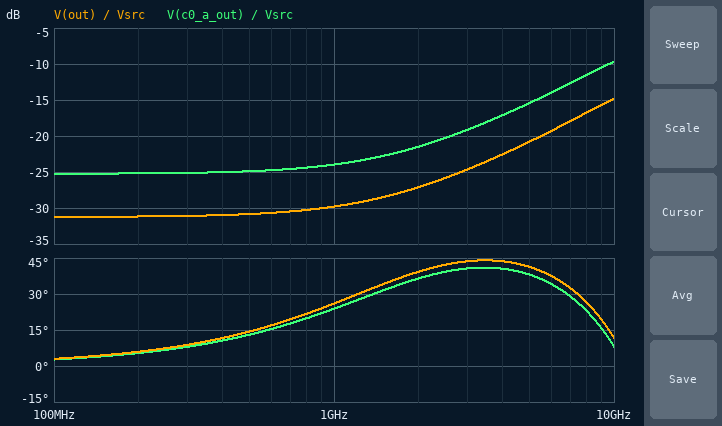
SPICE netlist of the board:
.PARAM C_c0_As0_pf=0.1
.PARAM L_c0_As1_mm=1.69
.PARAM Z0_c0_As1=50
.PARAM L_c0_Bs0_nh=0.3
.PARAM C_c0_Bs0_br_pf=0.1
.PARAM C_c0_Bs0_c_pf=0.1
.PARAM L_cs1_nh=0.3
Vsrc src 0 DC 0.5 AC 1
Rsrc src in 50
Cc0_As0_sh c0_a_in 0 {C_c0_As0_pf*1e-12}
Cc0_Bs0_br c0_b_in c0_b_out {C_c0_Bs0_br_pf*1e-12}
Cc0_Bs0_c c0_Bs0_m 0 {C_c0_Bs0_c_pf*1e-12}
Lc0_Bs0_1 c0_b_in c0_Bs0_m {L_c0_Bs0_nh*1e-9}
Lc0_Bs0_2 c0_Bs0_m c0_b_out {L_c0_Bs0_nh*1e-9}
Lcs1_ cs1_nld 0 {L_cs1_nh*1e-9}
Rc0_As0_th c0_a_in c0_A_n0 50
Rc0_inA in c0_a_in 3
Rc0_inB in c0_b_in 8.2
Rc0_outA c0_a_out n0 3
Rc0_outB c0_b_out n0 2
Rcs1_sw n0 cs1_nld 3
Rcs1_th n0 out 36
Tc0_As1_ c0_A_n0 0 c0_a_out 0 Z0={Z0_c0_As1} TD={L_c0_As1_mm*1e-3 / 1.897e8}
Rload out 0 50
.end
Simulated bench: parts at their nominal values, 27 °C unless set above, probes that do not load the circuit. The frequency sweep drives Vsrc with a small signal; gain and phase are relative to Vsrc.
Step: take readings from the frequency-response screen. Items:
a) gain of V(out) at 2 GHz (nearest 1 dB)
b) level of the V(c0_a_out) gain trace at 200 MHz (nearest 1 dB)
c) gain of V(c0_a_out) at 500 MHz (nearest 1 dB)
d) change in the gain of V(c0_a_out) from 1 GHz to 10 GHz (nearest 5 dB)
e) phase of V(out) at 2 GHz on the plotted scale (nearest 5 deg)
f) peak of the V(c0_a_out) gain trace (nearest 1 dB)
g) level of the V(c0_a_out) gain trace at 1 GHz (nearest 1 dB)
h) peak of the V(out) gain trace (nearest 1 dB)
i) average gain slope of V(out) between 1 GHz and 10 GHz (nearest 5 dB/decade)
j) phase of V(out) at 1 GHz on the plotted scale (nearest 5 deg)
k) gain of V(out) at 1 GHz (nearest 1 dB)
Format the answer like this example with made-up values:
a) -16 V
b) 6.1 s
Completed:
a) -27 dB
b) -25 dB
c) -25 dB
d) 15 dB
e) 40 deg
f) -10 dB
g) -24 dB
h) -15 dB
i) 15 dB/decade
j) 25 deg
k) -30 dB
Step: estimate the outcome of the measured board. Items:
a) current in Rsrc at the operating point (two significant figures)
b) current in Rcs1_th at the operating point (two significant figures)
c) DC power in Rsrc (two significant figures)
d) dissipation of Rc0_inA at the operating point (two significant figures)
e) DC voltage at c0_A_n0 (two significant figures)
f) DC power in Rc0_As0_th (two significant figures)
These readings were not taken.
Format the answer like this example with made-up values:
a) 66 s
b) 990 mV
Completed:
a) 8.1 mA
b) 270 µA
c) 3.3 mW
d) 4.7 µW
e) 27 mV
f) 78 µW
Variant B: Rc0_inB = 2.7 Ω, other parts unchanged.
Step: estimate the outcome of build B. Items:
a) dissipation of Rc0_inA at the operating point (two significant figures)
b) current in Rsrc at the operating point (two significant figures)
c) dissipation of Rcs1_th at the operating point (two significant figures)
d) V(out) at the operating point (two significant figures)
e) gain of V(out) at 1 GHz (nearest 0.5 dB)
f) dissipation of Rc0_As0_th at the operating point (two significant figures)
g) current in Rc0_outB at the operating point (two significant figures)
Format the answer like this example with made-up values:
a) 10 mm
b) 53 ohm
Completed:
a) 1.4 µW
b) 8.7 mA
c) 3.1 µW
d) 15 mV
e) -29.0 dB
f) 23 µW
g) 8.1 mA
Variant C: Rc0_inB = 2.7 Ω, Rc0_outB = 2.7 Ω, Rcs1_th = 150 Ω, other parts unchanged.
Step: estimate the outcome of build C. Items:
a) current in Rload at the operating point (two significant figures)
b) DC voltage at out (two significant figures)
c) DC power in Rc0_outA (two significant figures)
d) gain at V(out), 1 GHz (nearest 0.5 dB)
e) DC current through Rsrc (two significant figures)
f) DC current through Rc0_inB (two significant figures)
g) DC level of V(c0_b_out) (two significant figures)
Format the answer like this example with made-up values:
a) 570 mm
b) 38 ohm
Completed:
a) 130 µA
b) 6.4 mV
c) 1.7 µW
d) -36.5 dB
e) 8.6 mA
f) 7.9 mA
g) 47 mV
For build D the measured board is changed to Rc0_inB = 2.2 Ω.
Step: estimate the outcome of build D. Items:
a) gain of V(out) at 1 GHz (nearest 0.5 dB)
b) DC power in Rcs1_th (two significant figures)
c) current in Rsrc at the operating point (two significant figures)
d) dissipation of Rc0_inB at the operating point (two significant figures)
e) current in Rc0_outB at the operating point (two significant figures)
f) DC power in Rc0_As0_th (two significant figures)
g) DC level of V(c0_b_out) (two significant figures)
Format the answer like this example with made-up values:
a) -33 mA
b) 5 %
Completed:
a) -29.0 dB
b) 3.2 µW
c) 8.8 mA
d) 150 µW
e) 8.2 mA
f) 19 µW
g) 42 mV
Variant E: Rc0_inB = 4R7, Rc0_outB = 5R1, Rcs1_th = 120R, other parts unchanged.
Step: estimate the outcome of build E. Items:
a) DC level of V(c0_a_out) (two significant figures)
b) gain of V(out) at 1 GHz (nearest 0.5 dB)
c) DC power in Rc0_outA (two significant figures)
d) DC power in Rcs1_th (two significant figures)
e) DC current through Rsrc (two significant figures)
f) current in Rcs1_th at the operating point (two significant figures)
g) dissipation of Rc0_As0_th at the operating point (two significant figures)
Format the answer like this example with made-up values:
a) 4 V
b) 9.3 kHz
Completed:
a) 28 mV
b) -35.5 dB
c) 4.4 µW
d) 2.4 µW
e) 8.2 mA
f) 140 µA
g) 74 µW
